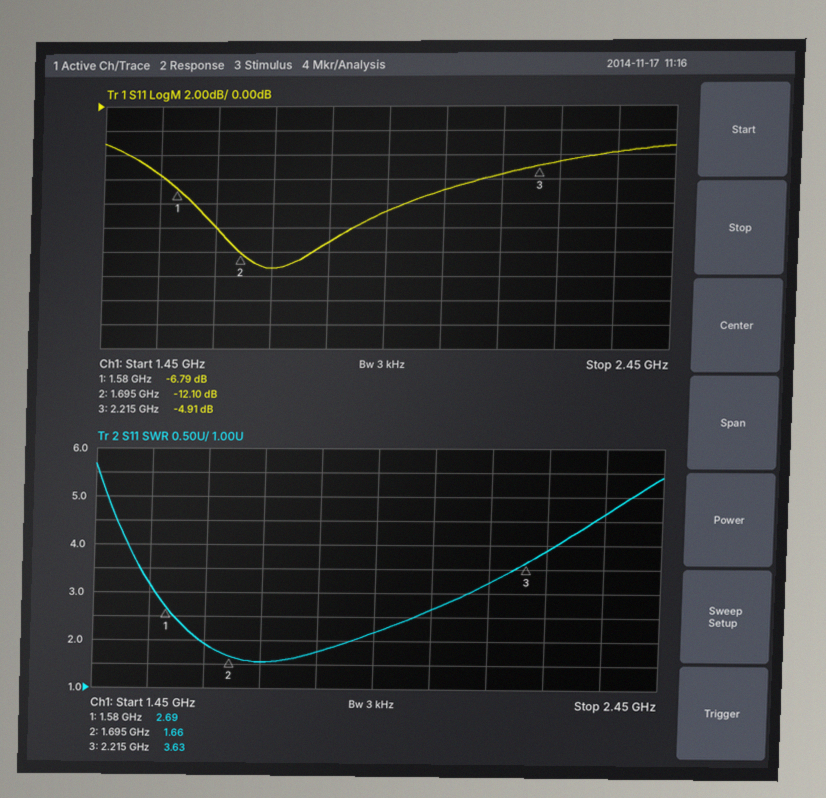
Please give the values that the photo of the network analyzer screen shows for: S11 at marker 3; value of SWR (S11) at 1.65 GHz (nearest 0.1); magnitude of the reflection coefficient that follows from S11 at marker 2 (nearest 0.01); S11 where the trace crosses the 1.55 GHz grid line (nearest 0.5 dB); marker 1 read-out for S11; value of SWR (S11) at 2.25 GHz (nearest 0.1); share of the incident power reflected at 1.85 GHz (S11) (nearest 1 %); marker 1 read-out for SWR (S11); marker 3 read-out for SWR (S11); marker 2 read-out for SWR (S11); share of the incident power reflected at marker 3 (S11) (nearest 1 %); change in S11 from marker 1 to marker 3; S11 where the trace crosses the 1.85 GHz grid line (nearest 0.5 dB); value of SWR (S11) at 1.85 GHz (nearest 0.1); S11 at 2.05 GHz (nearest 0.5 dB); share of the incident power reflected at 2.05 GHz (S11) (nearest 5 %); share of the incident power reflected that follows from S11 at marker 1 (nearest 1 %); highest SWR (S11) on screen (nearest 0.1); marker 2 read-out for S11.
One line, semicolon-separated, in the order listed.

-4.91 dB; 1.9; 0.25; -5.5 dB; -6.79 dB; 3.9; 8 %; 2.69; 3.63; 1.66; 32 %; 1.88 dB; -11.0 dB; 1.8; -7.0 dB; 20 %; 21 %; 5.7; -12.10 dB
